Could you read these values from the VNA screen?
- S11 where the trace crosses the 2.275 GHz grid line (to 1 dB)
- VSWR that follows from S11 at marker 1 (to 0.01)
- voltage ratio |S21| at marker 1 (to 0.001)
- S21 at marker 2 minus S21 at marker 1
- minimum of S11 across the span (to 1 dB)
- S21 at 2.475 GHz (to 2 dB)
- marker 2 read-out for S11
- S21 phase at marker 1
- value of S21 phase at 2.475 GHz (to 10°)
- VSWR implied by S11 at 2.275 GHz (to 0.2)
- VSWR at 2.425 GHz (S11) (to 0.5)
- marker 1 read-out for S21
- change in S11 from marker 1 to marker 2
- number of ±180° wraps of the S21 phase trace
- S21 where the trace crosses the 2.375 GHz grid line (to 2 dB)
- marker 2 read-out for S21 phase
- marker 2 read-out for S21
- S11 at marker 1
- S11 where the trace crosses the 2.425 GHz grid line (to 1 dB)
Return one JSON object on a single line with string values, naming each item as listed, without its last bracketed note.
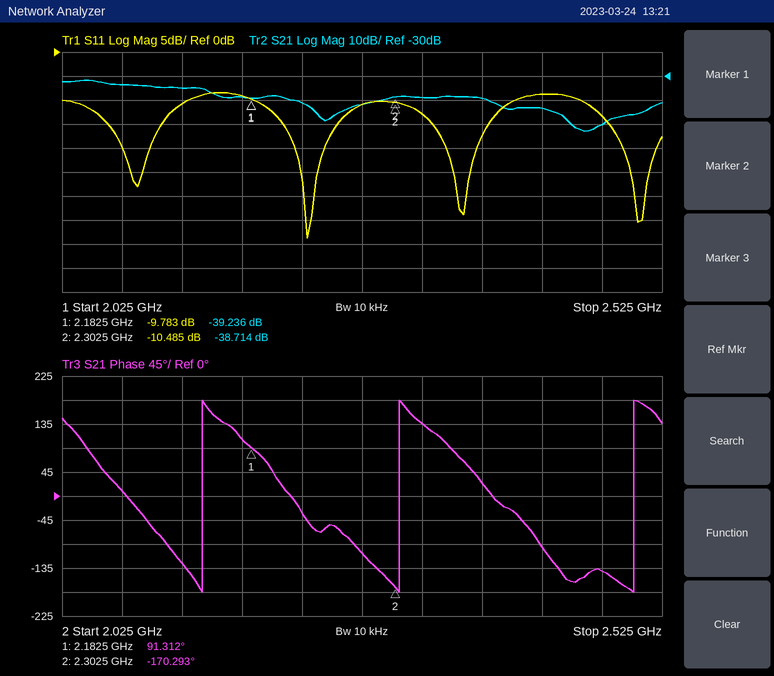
{"S11 where the trace crosses the 2.275 GHz grid line": "-11 dB", "VSWR that follows from S11 at marker 1": "1.96", "voltage ratio |S21| at marker 1": "0.011", "S21 at marker 2 minus S21 at marker 1": "0.522 dB", "minimum of S11 across the span": "-39 dB", "S21 at 2.475 GHz": "-50 dB", "marker 2 read-out for S11": "-10.485 dB", "S21 phase at marker 1": "91.312°", "value of S21 phase at 2.475 GHz": "-140°", "VSWR implied by S11 at 2.275 GHz": "1.8", "VSWR at 2.425 GHz (S11)": "2.0", "marker 1 read-out for S21": "-39.236 dB", "change in S11 from marker 1 to marker 2": "-0.702 dB", "number of ±180° wraps of the S21 phase trace": "3", "S21 where the trace crosses the 2.375 GHz grid line": "-40 dB", "marker 2 read-out for S21 phase": "-170.293°", "marker 2 read-out for S21": "-38.714 dB", "S11 at marker 1": "-9.783 dB", "S11 where the trace crosses the 2.425 GHz grid line": "-9 dB"}
